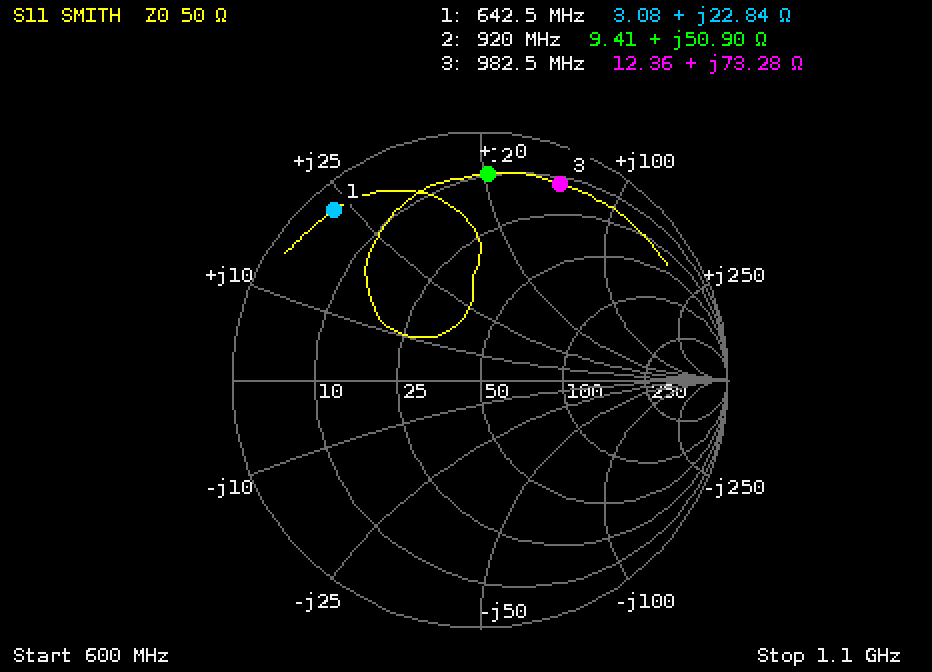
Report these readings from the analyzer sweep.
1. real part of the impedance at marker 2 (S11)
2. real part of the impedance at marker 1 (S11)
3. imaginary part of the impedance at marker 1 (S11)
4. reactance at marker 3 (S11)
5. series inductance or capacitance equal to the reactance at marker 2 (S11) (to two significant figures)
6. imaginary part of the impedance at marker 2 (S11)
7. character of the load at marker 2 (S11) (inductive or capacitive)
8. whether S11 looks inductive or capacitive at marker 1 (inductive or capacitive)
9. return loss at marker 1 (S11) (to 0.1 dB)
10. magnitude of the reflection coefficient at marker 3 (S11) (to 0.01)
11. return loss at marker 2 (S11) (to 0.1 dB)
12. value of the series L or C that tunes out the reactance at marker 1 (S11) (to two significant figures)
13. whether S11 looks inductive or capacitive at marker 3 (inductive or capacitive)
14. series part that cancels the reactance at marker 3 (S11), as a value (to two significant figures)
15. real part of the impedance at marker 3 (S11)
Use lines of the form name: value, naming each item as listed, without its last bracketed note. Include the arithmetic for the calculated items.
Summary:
real part of the impedance at marker 2: 9.41 Ω
real part of the impedance at marker 1: 3.08 Ω
imaginary part of the impedance at marker 1: +22.84 Ω
reactance at marker 3: +73.28 Ω
series inductance or capacitance equal to the reactance at marker 2 (S11): L = 50.9 Ω/(2π × 920 MHz) ≈ 8.8 nH
imaginary part of the impedance at marker 2: +50.90 Ω
character of the load at marker 2 (S11): inductive
whether S11 looks inductive or capacitive at marker 1: inductive
return loss at marker 1 (S11): 0.9 dB
magnitude of the reflection coefficient at marker 3 (S11): 0.86
return loss at marker 2 (S11): 1.6 dB
value of the series L or C that tunes out the reactance at marker 1 (S11): C = 1/(2π × 642.5 MHz × 22.84 Ω) ≈ 11 pF
whether S11 looks inductive or capacitive at marker 3: inductive
series part that cancels the reactance at marker 3 (S11), as a value: C = 1/(2π × 982.5 MHz × 73.28 Ω) ≈ 2.2 pF
real part of the impedance at marker 3: 12.36 Ω
